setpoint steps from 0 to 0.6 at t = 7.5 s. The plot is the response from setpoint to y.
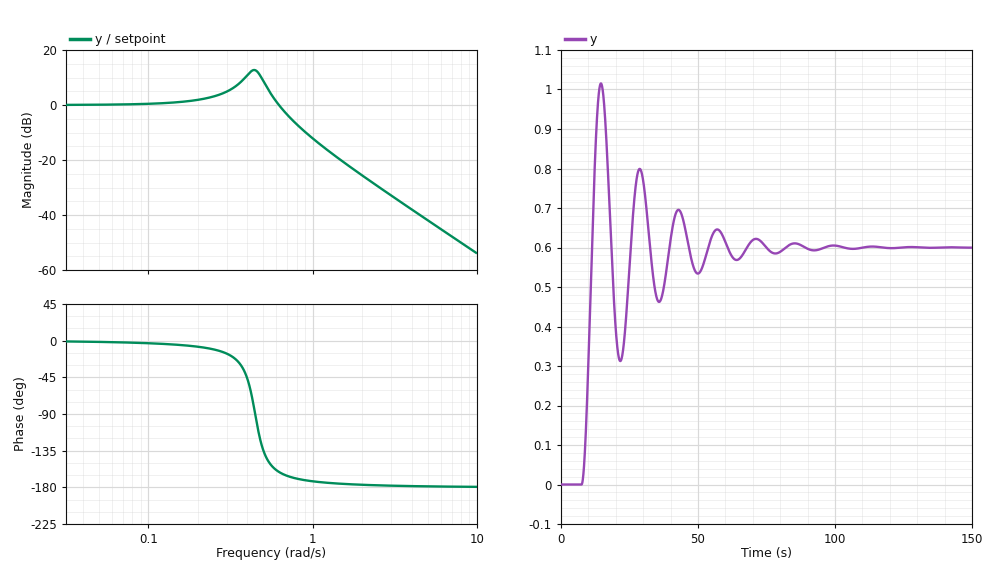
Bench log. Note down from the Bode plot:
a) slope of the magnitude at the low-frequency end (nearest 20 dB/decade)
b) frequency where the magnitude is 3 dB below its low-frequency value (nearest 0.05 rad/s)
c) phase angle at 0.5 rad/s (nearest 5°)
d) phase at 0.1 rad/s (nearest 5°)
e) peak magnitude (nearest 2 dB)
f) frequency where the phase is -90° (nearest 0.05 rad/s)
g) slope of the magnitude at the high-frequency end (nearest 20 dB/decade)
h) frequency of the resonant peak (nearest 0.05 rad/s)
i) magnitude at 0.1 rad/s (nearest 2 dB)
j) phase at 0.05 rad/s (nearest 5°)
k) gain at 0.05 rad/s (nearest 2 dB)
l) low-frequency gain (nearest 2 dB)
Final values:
0 dB/decade
0.70 rad/s
-135°
-5°
12 dB
0.45 rad/s
-40 dB/decade
0.45 rad/s
0 dB
0°
0 dB
0 dB
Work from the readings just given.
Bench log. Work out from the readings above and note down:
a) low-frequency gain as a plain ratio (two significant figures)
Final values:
1.0
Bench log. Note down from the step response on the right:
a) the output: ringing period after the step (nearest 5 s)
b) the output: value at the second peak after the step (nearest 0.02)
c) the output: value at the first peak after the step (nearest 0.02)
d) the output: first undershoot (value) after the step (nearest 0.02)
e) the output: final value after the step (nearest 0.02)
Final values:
15 s
0.80
1.02
0.32
0.60
